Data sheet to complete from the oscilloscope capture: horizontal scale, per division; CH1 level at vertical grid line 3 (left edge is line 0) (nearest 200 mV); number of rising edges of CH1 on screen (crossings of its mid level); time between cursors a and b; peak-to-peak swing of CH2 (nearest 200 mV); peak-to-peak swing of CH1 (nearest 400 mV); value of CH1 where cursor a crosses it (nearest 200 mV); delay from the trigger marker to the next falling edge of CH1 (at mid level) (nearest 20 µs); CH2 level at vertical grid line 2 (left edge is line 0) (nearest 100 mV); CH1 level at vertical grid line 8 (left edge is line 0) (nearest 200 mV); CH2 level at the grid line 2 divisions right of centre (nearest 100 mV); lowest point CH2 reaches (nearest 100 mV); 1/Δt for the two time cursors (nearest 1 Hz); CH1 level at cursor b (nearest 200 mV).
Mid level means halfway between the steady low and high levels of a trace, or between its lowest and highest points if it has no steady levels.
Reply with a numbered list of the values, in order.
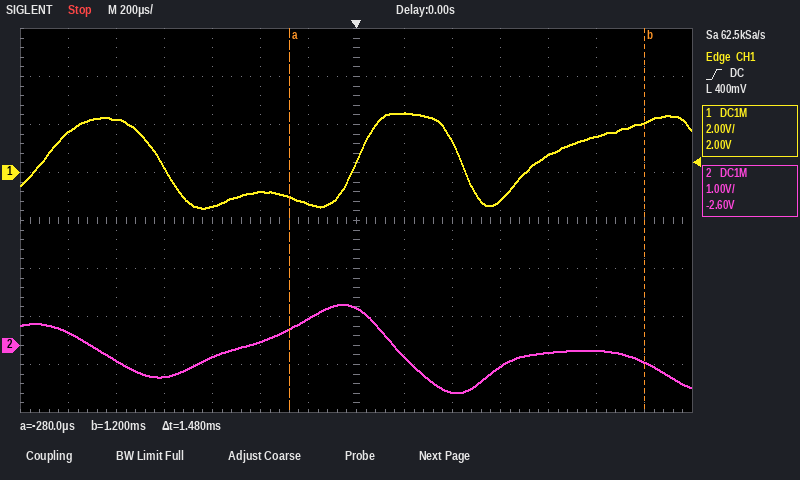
1. 200 µs
2. 200 mV
3. 3
4. 1.48 ms
5. 1.8 V
6. 4.0 V
7. -1.0 V
8. 440 µs
9. -300 mV
10. 2.4 V
11. -1.0 V
12. -1.0 V
13. 676 Hz
14. 2.0 V
